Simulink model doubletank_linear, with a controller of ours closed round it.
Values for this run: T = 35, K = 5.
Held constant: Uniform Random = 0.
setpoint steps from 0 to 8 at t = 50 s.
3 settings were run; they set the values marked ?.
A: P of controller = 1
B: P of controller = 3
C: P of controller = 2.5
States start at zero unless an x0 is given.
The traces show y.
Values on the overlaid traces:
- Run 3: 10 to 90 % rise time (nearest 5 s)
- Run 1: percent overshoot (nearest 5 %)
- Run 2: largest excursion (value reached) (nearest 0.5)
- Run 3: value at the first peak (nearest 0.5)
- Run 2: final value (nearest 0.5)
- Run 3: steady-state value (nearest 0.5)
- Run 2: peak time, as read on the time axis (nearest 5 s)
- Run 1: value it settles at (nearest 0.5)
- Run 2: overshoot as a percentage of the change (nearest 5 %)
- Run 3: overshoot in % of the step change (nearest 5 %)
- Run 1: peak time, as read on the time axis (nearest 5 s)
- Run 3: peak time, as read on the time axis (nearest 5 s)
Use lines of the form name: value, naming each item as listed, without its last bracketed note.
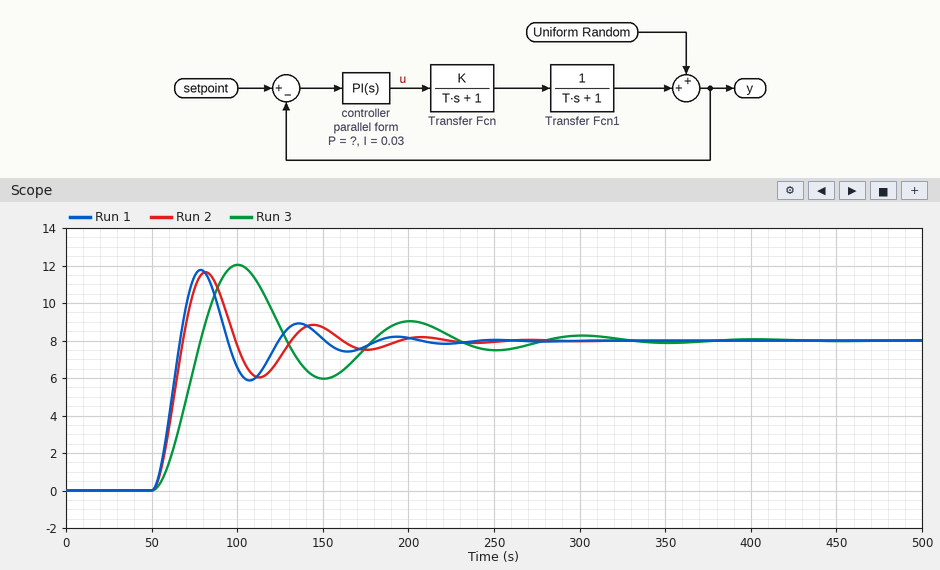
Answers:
Run 3: 10 to 90 % rise time: 20 s
Run 1: percent overshoot: 45 %
Run 2: largest excursion (value reached): 11.5
Run 3: value at the first peak: 12.0
Run 2: final value: 8.0
Run 3: steady-state value: 8.0
Run 2: peak time, as read on the time axis: 80 s
Run 1: value it settles at: 8.0
Run 2: overshoot as a percentage of the change: 45 %
Run 3: overshoot in % of the step change: 50 %
Run 1: peak time, as read on the time axis: 80 s
Run 3: peak time, as read on the time axis: 100 s
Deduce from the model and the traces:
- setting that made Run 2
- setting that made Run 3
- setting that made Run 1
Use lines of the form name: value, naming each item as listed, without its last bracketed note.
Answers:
setting that made Run 2: C
setting that made Run 3: A
setting that made Run 1: B
